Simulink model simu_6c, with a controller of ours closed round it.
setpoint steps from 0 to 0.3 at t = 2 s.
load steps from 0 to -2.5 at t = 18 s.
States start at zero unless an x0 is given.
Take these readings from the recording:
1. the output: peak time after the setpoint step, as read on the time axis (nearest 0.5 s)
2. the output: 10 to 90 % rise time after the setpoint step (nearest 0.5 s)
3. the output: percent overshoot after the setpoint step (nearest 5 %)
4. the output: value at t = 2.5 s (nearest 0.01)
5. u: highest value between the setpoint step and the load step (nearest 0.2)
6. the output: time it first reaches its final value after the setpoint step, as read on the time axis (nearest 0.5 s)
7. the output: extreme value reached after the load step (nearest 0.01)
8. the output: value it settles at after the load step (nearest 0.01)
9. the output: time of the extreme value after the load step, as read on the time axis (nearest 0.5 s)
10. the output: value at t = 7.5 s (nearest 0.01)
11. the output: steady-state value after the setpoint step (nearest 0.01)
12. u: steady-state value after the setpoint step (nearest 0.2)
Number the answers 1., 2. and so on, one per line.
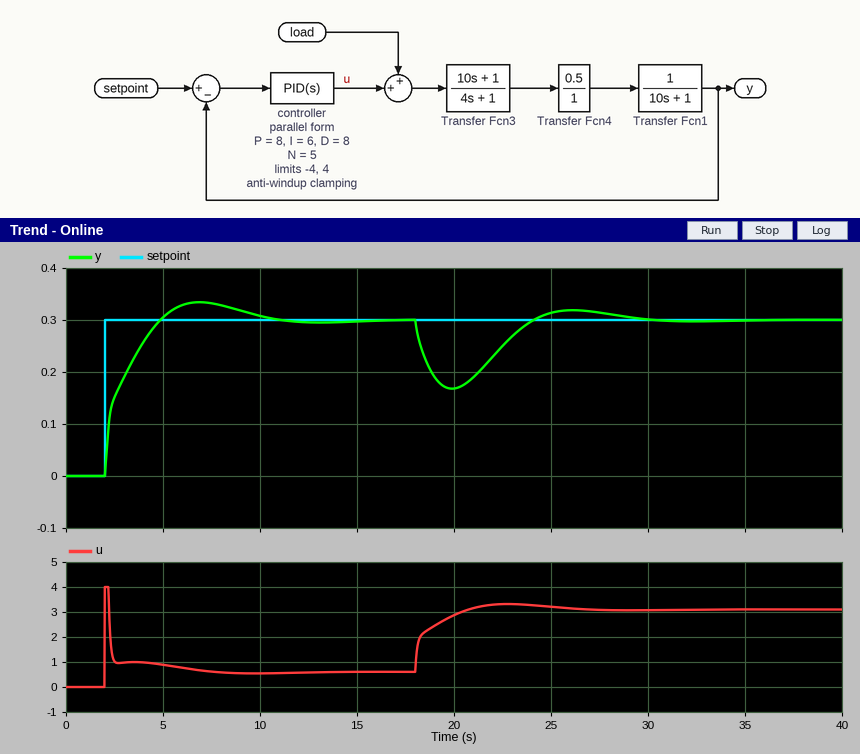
1. 7.0 s
2. 2.0 s
3. 10 %
4. 0.15
5. 4.0
6. 5.0 s
7. 0.17
8. 0.30
9. 20.0 s
10. 0.33
11. 0.30
12. 0.6
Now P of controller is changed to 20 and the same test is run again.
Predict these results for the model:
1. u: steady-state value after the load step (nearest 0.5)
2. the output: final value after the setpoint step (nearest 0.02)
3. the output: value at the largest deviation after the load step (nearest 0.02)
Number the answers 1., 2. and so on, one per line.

1. 3.0
2. 0.30
3. 0.22
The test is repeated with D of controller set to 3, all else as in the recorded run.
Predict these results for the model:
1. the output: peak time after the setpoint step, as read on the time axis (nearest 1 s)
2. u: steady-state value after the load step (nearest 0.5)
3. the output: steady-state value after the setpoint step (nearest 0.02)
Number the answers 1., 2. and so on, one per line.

1. 6 s
2. 3.0
3. 0.30
